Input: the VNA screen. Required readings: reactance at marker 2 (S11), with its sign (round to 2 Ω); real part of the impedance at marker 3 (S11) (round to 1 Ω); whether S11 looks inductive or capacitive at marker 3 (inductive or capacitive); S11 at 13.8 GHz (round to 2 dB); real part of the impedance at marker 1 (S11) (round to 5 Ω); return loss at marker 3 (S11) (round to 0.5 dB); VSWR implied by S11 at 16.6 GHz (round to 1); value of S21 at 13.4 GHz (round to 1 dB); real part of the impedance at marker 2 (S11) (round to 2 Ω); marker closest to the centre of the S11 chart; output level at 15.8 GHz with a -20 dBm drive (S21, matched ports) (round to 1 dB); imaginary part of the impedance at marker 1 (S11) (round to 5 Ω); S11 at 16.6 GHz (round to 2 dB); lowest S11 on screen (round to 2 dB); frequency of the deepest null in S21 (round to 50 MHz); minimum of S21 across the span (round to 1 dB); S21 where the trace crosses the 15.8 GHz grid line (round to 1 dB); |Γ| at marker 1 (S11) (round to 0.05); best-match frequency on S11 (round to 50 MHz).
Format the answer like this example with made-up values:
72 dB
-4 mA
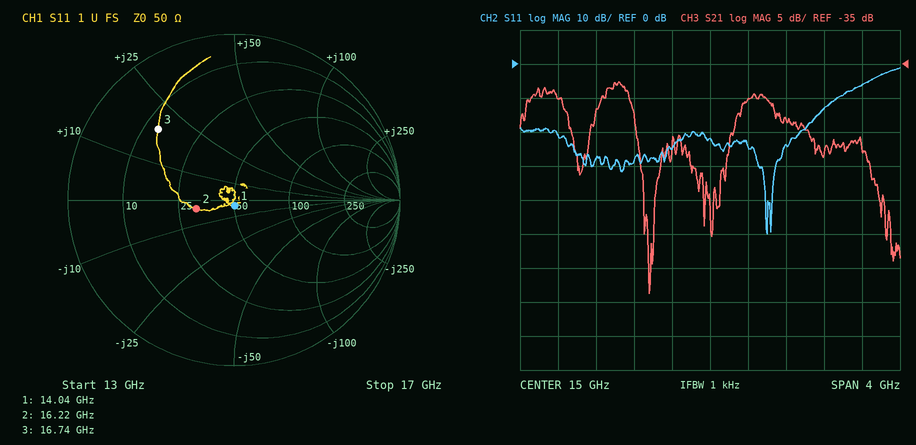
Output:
-4 Ω
13 Ω
inductive
-28 dB
50 Ω
4.0 dB
3
-40 dB
32 Ω
marker 1
-63 dBm
-5 Ω
-6 dB
-50 dB
14.35 GHz
-69 dB
-43 dB
0.05
15.60 GHz
